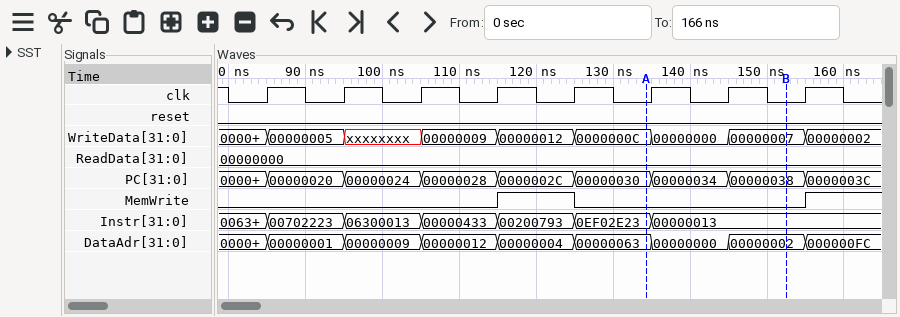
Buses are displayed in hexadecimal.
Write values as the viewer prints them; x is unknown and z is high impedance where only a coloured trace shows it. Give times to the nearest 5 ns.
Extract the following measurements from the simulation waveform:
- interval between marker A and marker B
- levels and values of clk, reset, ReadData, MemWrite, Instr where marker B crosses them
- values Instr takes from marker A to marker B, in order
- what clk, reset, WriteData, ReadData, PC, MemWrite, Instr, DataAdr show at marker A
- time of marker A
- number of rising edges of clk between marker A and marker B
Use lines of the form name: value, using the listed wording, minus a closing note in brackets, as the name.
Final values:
interval between marker A and marker B: 20 ns
levels and values of clk, reset, ReadData, MemWrite, Instr where marker B crosses them: clk=0, reset=0, ReadData=00000000, MemWrite=0, Instr=00000013
values Instr takes from marker A to marker B, in order: 0EF02E23, 00000013
what clk, reset, WriteData, ReadData, PC, MemWrite, Instr, DataAdr show at marker A: clk=0, reset=0, WriteData=0000000C, ReadData=00000000, PC=00000030, MemWrite=0, Instr=0EF02E23, DataAdr=00000063
time of marker A: 135 ns
number of rising edges of clk between marker A and marker B: 2
